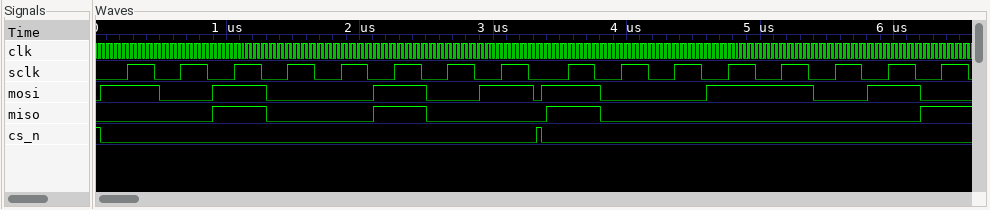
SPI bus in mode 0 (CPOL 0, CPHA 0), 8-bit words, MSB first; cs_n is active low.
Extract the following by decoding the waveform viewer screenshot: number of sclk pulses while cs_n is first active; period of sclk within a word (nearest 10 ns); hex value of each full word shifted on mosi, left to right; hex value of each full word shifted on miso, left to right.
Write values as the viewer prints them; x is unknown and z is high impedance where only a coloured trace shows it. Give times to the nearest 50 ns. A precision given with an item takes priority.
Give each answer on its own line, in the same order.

8
400 ns
A5, 9A
24, 81
